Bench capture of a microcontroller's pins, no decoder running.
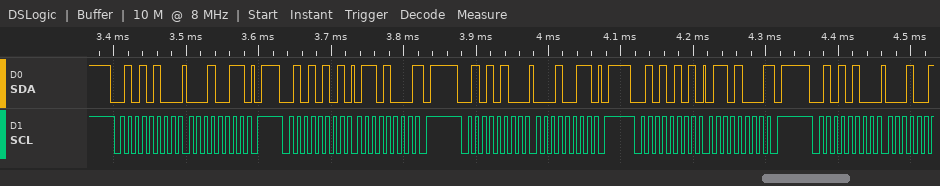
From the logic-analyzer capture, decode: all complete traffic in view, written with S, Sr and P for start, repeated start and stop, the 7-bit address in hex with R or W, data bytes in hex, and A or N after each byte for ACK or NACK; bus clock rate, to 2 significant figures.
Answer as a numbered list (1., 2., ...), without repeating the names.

1. S 2AW A 13 A P S 2AR A 68 N P S 2AW A 13 A P S 2AR A 68 N P S 2AW A
2. 100 kHz
